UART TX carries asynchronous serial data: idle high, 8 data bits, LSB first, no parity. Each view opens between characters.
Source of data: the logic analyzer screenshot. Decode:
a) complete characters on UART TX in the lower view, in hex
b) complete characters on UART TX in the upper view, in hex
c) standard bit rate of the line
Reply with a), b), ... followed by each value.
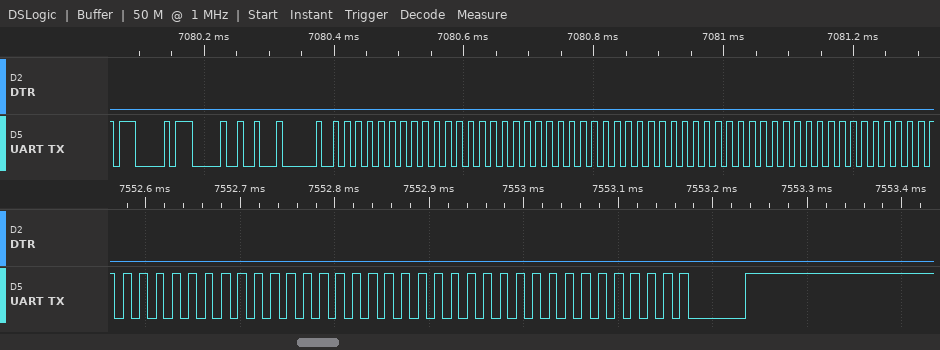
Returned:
a) 55, 55, 55, 55, 55, 55, 55, C0
b) 07, 07, 12, 20, 55, 55, 55, 55, 55, 55, 55, 55, 55, 55
c) 115200 baud
